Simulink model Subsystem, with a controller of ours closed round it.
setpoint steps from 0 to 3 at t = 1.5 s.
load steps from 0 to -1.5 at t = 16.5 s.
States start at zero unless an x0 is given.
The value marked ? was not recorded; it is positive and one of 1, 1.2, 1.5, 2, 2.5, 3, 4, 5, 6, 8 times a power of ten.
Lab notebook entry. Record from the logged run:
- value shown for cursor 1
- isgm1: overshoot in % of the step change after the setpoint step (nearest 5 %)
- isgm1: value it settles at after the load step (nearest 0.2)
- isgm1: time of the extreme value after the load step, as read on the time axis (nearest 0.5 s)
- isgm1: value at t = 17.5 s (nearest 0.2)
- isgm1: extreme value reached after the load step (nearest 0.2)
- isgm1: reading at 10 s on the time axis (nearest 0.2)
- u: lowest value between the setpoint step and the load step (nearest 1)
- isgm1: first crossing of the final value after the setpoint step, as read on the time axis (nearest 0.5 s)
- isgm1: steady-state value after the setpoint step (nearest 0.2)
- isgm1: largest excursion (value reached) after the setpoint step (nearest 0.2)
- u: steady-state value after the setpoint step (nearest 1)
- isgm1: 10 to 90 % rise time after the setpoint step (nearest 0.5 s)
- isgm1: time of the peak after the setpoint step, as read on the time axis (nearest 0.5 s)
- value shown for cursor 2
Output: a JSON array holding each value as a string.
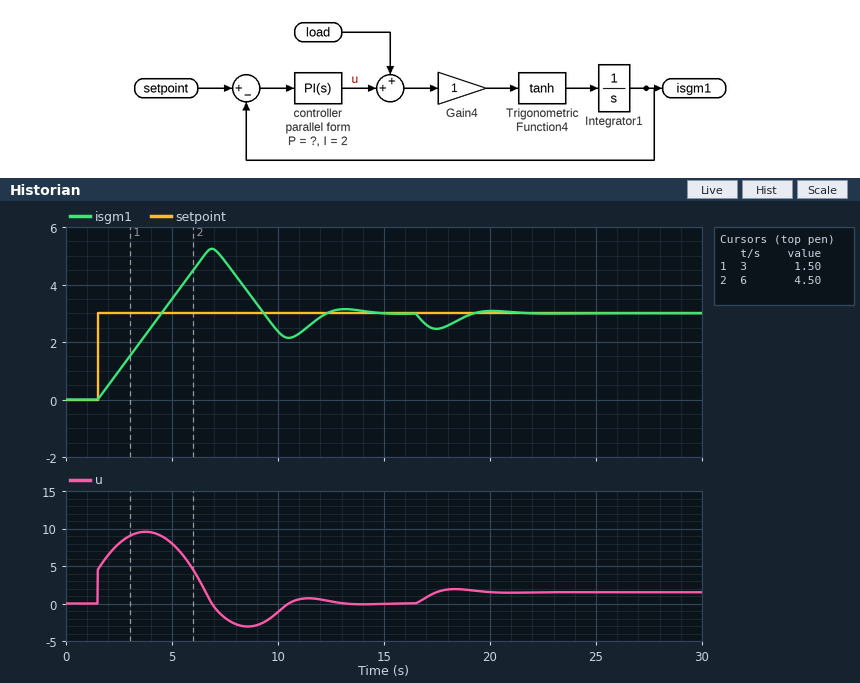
["1.50", "75 %", "3.0", "17.5 s", "2.4", "2.4", "2.4", "-3", "4.5 s", "3.0", "5.2", "0", "2.5 s", "7.0 s", "4.50"]
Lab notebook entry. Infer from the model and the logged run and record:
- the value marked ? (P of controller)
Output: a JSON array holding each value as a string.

["1.5"]
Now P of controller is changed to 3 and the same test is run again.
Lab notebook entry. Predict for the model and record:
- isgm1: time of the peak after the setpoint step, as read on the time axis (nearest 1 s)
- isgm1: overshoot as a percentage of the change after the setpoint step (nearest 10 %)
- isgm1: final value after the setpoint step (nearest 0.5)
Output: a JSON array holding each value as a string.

["6 s", "60 %", "3.0"]
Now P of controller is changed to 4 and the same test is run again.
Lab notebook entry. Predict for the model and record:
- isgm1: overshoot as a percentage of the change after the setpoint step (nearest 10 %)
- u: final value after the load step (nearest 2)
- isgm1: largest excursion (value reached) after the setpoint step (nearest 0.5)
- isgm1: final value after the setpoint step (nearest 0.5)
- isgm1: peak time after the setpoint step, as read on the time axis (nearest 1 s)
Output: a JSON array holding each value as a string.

["50 %", "2", "4.5", "3.0", "6 s"]
